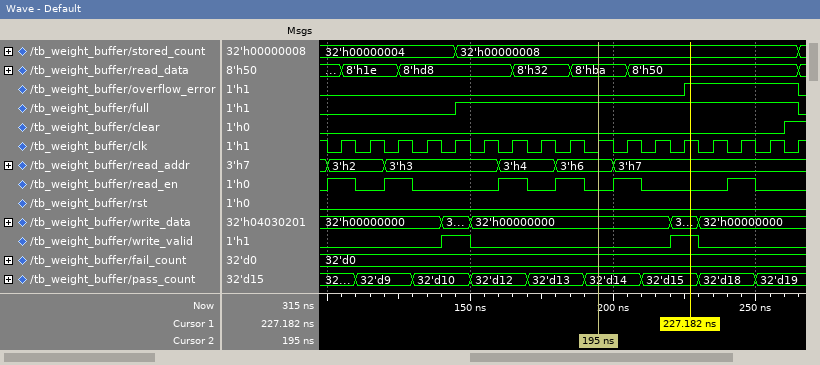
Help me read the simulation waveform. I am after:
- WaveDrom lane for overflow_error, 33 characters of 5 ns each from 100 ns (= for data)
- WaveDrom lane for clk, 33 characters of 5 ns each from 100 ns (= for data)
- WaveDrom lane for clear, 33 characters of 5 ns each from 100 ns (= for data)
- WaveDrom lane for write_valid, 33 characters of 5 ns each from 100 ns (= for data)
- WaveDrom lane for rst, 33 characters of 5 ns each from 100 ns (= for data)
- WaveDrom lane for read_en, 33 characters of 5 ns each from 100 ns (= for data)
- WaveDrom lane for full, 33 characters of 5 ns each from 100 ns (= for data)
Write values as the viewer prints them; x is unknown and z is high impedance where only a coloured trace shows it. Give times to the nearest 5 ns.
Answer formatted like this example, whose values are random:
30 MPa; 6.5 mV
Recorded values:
{name: 'overflow_error', wave: '0........................1.......'}; {name: 'clk', wave: '010101010101010101010101010101010'}; {name: 'clear', wave: '0...............................1'}; {name: 'write_valid', wave: '0.......1.0.............1.0......'}; {name: 'rst', wave: '0................................'}; {name: 'read_en', wave: '1.0.1.0.....1.0.1.0.1.0.....1.0..'}; {name: 'full', wave: '0........1.......................'}
